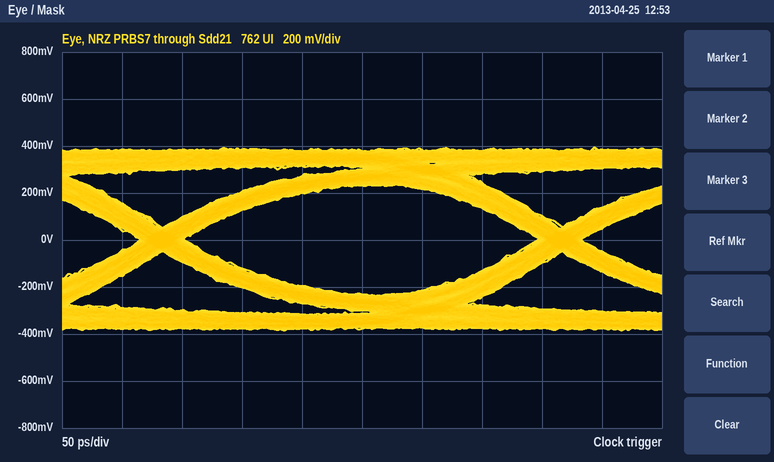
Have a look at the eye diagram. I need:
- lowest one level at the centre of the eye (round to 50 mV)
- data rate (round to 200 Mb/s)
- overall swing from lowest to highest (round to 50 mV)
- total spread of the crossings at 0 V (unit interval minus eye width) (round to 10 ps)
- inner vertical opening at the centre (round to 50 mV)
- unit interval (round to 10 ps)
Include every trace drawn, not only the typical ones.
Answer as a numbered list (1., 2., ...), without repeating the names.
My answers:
1. 250 mV
2. 3.0 Gb/s
3. 800 mV
4. 40 ps
5. 450 mV
6. 330 ps
